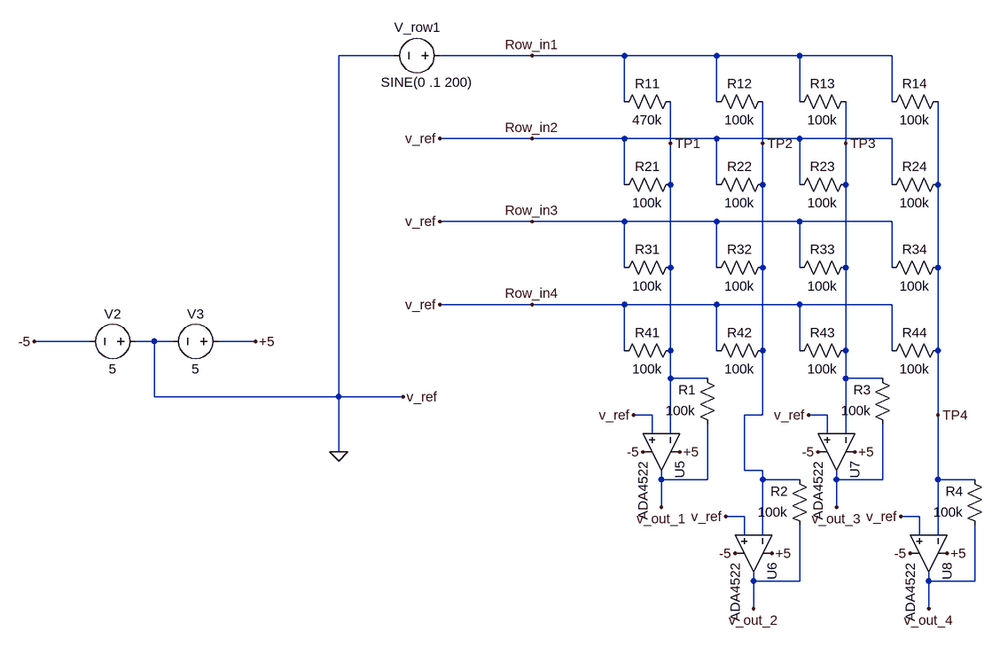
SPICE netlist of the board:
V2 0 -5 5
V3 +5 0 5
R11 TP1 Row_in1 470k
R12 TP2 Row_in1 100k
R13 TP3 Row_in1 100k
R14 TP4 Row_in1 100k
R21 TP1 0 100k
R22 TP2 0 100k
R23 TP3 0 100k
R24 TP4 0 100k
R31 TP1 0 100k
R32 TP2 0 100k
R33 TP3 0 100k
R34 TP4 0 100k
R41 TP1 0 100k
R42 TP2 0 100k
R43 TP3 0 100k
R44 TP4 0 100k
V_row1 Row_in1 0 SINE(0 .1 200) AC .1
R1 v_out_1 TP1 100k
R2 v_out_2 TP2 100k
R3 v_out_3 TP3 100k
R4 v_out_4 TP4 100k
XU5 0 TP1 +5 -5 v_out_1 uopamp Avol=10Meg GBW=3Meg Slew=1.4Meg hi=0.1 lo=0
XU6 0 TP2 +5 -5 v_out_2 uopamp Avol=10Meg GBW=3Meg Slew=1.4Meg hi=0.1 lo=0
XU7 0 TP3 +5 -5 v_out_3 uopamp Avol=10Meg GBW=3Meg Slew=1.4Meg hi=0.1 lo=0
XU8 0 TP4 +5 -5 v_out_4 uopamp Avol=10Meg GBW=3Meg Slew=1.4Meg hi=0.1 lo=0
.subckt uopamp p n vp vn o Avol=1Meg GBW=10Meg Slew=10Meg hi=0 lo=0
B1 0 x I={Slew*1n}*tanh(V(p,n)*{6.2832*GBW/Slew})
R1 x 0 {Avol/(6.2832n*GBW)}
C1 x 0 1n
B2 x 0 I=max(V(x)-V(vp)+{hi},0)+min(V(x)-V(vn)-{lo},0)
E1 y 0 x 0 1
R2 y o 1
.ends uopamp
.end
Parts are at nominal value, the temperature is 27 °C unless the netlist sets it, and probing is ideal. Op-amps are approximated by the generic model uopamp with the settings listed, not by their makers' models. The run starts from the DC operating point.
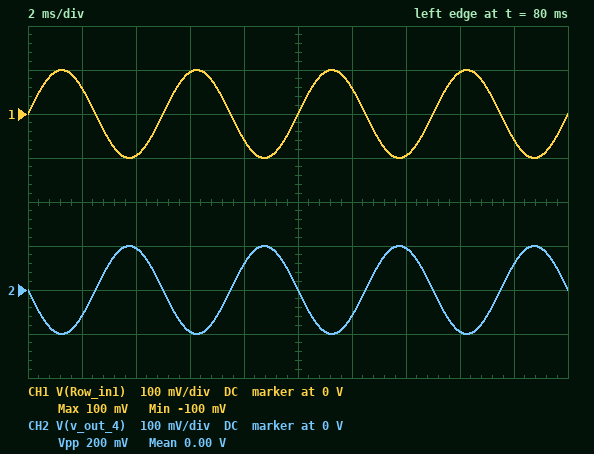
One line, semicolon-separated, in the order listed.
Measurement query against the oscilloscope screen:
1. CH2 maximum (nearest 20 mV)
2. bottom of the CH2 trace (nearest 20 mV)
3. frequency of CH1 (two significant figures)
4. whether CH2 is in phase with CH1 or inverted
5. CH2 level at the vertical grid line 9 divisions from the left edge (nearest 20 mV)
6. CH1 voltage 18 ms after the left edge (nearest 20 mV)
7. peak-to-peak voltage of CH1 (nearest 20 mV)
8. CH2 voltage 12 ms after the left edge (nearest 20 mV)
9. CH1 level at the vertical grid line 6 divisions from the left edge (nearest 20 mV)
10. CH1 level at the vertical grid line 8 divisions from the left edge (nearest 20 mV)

100 mV; -100 mV; 200 Hz; inverted; 60 mV; -60 mV; 200 mV; -60 mV; 60 mV; 100 mV
